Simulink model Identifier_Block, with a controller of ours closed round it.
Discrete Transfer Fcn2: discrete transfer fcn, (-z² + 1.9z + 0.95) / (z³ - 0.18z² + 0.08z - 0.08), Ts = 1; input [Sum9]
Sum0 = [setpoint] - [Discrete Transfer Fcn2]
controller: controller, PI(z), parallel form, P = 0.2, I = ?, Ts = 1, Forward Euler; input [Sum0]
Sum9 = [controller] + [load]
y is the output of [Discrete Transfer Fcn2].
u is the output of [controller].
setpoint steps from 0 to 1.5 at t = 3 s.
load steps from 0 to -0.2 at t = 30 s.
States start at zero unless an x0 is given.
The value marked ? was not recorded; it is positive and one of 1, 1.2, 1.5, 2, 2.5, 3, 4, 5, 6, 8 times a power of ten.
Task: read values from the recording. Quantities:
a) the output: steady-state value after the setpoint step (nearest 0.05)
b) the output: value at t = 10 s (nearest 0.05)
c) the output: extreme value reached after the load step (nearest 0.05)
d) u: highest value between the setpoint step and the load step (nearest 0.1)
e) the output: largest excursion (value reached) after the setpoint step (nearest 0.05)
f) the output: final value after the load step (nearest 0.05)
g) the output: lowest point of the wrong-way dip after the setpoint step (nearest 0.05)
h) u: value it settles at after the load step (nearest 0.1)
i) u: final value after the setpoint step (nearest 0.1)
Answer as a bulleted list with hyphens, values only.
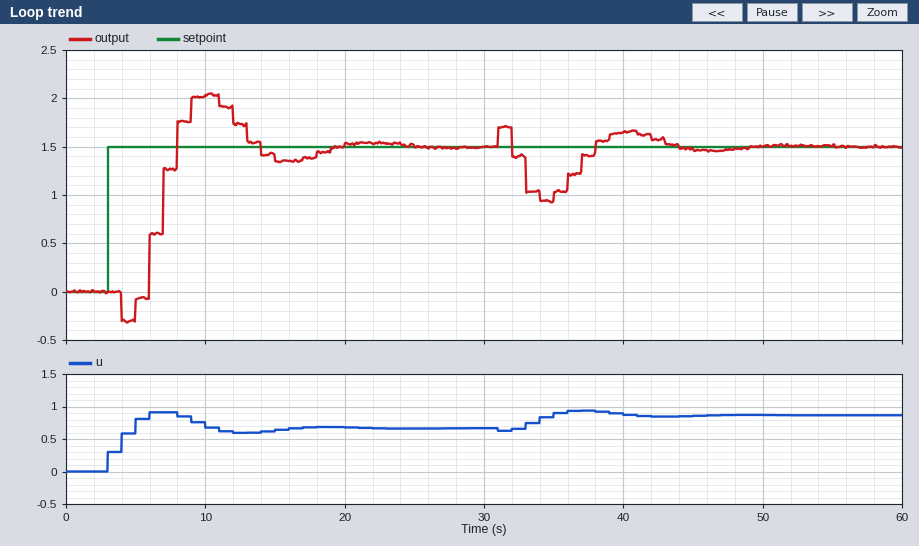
- 1.50
- 2.05
- 0.95
- 0.9
- 2.05
- 1.50
- -0.30
- 0.9
- 0.7
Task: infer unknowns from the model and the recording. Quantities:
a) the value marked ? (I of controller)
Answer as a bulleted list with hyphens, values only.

- 0.15
